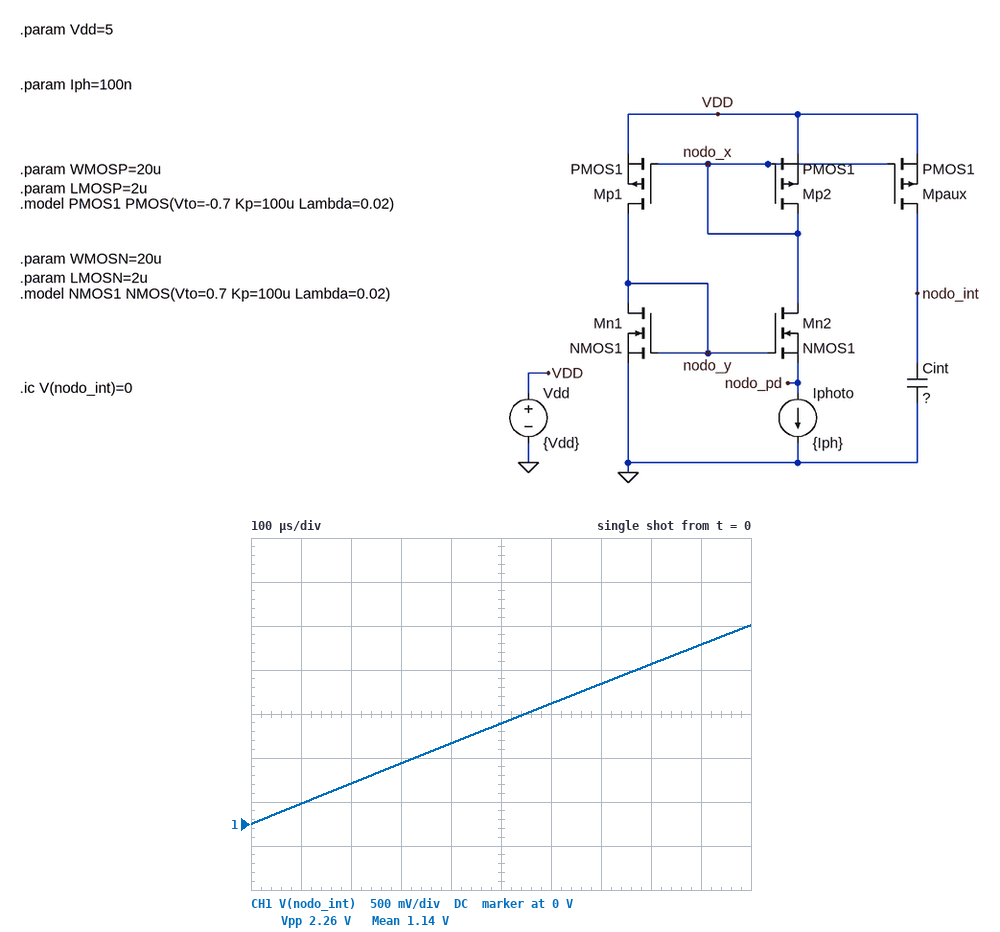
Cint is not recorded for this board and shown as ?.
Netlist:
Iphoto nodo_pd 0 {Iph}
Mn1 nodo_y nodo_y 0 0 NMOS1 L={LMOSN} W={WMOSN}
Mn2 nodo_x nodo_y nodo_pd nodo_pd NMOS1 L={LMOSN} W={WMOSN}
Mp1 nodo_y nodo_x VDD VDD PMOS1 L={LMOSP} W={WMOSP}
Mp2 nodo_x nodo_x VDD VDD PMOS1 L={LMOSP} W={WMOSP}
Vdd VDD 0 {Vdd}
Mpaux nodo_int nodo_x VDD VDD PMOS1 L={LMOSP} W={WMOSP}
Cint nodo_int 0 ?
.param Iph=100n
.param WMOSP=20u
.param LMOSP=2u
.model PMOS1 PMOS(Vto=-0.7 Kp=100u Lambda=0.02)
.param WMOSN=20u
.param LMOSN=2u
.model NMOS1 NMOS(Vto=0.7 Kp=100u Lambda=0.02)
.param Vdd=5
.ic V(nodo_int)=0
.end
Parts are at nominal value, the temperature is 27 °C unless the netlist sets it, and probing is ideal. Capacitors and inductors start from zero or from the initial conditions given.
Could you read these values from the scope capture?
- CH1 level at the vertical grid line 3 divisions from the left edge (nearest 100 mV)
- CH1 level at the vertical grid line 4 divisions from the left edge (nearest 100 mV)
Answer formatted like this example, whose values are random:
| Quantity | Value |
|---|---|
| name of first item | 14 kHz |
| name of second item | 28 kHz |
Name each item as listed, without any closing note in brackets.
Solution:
| Quantity | Value |
|---|---|
| CH1 level at the vertical grid line 3 divisions from the left edge | 700 mV |
| CH1 level at the vertical grid line 4 divisions from the left edge | 900 mV |
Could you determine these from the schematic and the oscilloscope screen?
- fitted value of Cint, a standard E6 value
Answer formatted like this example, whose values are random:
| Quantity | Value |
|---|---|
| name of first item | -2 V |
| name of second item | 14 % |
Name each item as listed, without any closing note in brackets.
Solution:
| Quantity | Value |
|---|---|
| fitted value of Cint, a standard E6 value | 47 pF |
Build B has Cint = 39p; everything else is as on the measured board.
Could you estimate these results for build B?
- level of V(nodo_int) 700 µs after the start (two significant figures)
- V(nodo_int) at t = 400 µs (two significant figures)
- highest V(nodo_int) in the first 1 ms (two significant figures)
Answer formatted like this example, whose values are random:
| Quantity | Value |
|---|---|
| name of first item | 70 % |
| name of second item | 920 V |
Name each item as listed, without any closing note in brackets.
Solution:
| Quantity | Value |
|---|---|
| level of V(nodo_int) 700 µs after the start | 1.9 V |
| V(nodo_int) at t = 400 µs | 1.1 V |
| highest V(nodo_int) in the first 1 ms | 2.7 V |
